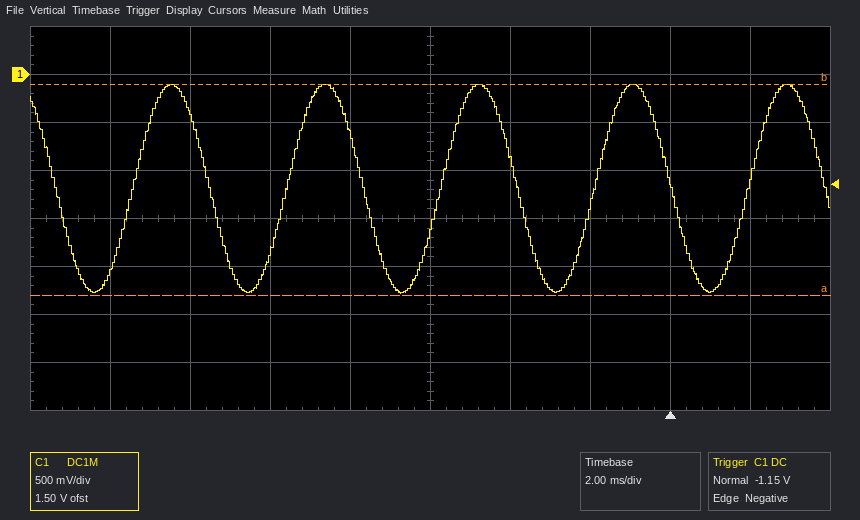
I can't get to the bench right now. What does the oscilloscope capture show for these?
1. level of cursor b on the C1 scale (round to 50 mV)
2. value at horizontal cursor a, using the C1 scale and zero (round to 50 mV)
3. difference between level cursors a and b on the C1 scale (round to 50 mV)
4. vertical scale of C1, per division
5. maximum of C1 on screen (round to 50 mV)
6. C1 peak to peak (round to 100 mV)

-100 mV
-2.30 V
2.20 V
500 mV
-100 mV
2.20 V
